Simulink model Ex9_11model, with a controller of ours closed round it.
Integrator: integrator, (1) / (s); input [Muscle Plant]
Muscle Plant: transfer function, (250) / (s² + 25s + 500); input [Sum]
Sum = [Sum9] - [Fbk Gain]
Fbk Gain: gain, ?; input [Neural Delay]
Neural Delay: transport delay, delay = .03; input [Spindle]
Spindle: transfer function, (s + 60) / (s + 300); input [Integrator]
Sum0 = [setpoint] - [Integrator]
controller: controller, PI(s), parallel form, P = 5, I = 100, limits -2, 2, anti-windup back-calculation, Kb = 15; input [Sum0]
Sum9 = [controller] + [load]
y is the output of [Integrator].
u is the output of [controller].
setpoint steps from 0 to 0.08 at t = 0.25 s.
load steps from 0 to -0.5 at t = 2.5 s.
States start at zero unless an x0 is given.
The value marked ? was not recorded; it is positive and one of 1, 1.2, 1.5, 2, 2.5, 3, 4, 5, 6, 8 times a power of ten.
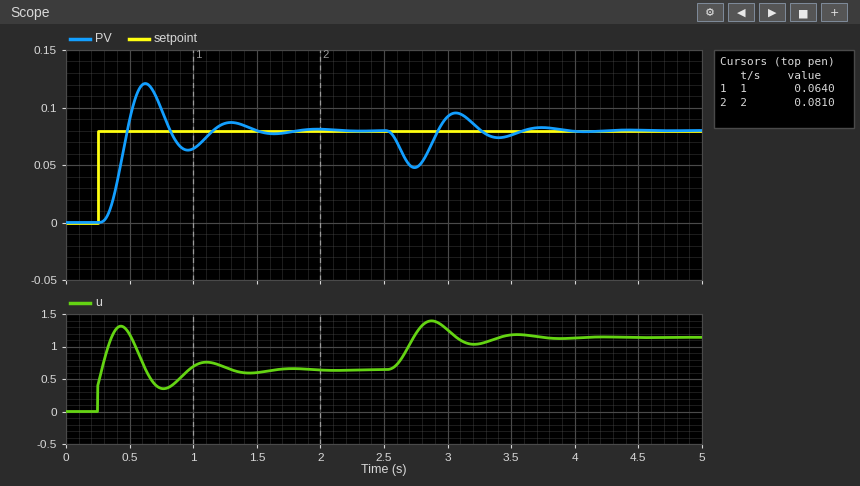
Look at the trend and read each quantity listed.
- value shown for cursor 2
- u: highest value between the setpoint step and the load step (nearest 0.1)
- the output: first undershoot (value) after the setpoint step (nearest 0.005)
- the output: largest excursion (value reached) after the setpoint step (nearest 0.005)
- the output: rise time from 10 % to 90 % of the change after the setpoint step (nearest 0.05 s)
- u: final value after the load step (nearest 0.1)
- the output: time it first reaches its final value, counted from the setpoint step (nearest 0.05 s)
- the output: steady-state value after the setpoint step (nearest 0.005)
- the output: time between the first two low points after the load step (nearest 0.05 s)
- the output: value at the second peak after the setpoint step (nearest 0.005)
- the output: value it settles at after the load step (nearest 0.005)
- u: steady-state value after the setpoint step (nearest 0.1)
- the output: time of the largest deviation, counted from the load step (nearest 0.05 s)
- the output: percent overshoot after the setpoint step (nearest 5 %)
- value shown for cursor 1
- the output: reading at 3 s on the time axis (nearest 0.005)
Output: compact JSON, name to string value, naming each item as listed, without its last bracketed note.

{"value shown for cursor 2": "0.0810", "u: highest value between the setpoint step and the load step": "1.3", "the output: first undershoot (value) after the setpoint step": "0.065", "the output: largest excursion (value reached) after the setpoint step": "0.120", "the output: rise time from 10 % to 90 % of the change after the setpoint step": "0.15 s", "u: final value after the load step": "1.1", "the output: time it first reaches its final value, counted from the setpoint step": "0.25 s", "the output: steady-state value after the setpoint step": "0.080", "the output: time between the first two low points after the load step": "0.65 s", "the output: value at the second peak after the setpoint step": "0.085", "the output: value it settles at after the load step": "0.080", "u: steady-state value after the setpoint step": "0.6", "the output: time of the largest deviation, counted from the load step": "0.25 s", "the output: percent overshoot after the setpoint step": "50 %", "value shown for cursor 1": "0.0640", "the output: reading at 3 s on the time axis": "0.090"}
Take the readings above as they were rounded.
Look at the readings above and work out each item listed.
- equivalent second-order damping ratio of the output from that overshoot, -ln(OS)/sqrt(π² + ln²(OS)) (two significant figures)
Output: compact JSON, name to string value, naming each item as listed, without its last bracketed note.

{"equivalent second-order damping ratio of the output from that overshoot, -ln(OS)/sqrt(π² + ln²(OS))": "0.22"}
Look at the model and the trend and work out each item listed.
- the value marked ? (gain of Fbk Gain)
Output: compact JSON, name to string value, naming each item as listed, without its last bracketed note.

{"the value marked ?": "40"}
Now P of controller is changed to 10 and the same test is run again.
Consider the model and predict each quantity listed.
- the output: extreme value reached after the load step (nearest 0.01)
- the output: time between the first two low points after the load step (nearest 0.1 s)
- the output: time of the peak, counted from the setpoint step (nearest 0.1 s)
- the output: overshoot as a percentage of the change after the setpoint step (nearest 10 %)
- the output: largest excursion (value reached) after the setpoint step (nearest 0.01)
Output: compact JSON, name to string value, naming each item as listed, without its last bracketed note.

{"the output: extreme value reached after the load step": "0.05", "the output: time between the first two low points after the load step": "0.5 s", "the output: time of the peak, counted from the setpoint step": "0.3 s", "the output: overshoot as a percentage of the change after the setpoint step": "40 %", "the output: largest excursion (value reached) after the setpoint step": "0.11"}
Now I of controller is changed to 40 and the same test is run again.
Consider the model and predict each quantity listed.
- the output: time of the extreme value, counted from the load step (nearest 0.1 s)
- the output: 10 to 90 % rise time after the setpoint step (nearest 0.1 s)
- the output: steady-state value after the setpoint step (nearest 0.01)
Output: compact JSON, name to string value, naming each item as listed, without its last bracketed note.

{"the output: time of the extreme value, counted from the load step": "0.3 s", "the output: 10 to 90 % rise time after the setpoint step": "0.3 s", "the output: steady-state value after the setpoint step": "0.08"}
